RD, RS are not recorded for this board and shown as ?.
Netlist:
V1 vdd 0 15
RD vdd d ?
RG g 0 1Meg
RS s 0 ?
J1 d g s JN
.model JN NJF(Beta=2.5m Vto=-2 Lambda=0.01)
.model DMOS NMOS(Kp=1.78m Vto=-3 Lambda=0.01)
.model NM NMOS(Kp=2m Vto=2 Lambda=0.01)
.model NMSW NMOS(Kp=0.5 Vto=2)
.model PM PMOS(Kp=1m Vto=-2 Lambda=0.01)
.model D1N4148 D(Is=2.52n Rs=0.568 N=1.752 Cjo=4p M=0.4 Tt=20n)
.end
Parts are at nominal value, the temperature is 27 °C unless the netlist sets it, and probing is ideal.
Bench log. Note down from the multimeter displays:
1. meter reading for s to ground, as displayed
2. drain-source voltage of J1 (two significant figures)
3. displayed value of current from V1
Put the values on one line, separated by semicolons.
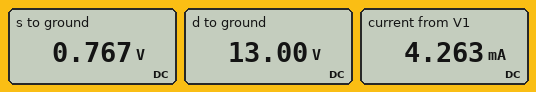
0.767 V; 12 V; 4.263 mA
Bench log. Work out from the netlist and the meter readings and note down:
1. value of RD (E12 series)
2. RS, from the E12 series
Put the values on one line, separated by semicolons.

470 Ω; 180 Ω
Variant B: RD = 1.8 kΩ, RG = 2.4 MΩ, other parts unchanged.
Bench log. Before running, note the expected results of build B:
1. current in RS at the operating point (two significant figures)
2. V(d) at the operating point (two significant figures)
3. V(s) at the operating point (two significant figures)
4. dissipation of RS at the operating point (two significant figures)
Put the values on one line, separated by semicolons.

4.2 mA; 7.5 V; 750 mV; 3.1 mW
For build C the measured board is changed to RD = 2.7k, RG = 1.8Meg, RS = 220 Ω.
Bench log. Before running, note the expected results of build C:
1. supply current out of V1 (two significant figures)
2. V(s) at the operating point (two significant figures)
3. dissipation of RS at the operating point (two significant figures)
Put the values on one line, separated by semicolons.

3.7 mA; 810 mV; 3.0 mW
